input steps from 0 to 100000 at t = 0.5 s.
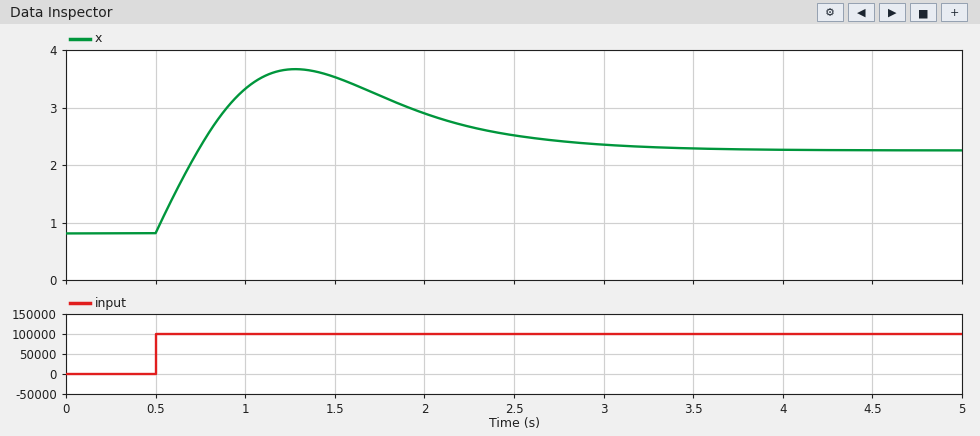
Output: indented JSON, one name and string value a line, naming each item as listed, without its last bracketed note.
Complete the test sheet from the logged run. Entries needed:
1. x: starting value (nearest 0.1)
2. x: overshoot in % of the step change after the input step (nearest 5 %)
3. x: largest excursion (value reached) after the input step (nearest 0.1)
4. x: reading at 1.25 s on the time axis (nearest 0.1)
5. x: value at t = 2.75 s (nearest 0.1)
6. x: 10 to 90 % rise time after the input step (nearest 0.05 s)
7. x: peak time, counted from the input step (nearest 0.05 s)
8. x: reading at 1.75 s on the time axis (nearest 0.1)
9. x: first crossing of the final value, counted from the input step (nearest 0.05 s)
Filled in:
{
  "x: starting value": "0.8",
  "x: overshoot in % of the step change after the input step": "100 %",
  "x: largest excursion (value reached) after the input step": "3.7",
  "x: reading at 1.25 s on the time axis": "3.7",
  "x: value at t = 2.75 s": "2.4",
  "x: 10 to 90 % rise time after the input step": "0.20 s",
  "x: peak time, counted from the input step": "0.80 s",
  "x: reading at 1.75 s on the time axis": "3.2",
  "x: first crossing of the final value, counted from the input step": "0.25 s"
}
